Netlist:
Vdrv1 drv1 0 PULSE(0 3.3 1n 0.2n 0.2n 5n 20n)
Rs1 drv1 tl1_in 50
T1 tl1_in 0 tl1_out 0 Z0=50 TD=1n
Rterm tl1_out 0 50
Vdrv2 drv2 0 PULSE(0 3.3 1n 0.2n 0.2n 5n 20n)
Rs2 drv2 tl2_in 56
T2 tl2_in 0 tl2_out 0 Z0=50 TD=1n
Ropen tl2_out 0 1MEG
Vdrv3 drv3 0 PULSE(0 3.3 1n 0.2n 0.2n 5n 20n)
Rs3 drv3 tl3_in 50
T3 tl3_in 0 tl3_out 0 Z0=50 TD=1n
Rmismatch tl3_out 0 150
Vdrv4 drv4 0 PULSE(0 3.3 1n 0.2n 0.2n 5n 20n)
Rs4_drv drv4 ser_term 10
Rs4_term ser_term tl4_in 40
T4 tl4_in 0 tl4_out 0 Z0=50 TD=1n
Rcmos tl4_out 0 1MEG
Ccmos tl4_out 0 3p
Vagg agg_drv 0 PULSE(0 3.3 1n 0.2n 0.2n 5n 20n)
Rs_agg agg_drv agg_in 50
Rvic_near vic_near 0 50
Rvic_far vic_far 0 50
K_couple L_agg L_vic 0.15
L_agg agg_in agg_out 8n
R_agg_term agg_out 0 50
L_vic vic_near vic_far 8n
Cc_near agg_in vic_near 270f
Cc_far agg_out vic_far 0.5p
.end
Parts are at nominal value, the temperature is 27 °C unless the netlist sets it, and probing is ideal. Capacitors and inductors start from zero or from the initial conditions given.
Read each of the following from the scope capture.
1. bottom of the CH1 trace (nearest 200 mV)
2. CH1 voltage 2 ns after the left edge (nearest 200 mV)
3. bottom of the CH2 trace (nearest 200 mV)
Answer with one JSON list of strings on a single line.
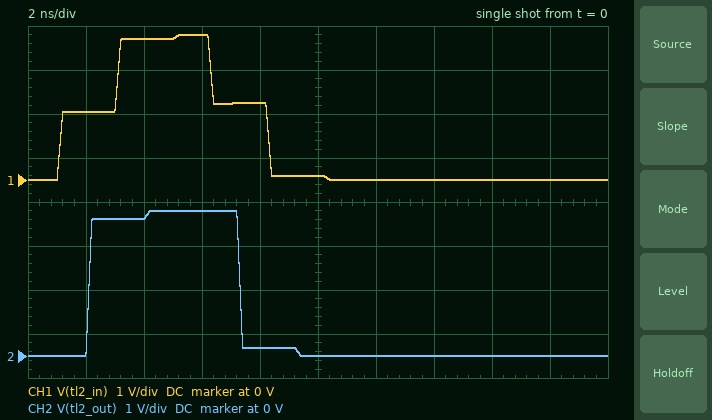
["0 V", "1.6 V", "0 V"]
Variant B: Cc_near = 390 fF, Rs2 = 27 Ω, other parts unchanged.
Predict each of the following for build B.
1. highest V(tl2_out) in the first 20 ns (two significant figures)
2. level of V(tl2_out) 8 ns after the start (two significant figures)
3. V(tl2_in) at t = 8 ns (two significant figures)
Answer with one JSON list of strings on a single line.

["4.3 V", "-900 mV", "1.2 V"]
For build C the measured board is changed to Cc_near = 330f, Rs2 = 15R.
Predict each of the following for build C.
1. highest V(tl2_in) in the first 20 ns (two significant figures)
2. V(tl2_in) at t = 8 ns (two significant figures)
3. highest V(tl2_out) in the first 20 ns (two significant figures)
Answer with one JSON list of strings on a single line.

["3.7 V", "880 mV", "5.1 V"]
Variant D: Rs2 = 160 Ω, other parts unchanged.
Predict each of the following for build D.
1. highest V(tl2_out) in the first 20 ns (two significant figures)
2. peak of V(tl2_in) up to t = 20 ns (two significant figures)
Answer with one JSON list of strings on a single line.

["2.8 V", "2.6 V"]
